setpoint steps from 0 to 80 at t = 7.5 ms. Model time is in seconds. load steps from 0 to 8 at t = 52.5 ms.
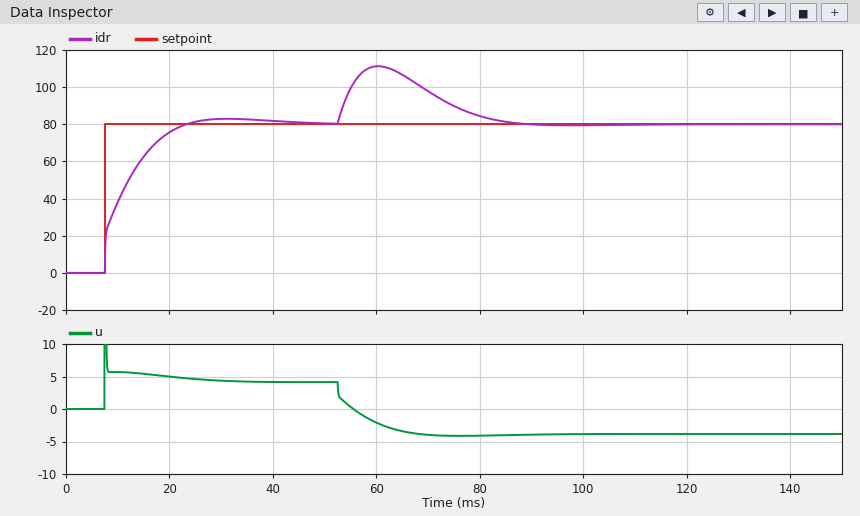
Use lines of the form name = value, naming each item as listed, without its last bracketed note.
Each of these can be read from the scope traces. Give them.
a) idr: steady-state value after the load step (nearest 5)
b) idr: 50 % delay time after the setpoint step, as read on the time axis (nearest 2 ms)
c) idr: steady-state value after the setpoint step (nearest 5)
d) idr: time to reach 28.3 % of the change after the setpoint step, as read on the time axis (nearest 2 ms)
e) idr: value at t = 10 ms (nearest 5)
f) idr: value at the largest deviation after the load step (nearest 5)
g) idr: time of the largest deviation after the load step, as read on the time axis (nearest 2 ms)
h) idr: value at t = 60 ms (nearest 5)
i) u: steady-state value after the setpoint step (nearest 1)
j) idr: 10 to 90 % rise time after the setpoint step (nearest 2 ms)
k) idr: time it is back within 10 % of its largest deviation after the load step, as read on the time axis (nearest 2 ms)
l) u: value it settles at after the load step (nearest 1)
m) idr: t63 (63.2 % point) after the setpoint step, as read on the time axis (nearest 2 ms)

idr: steady-state value after the load step = 80
idr: 50 % delay time after the setpoint step, as read on the time axis = 10 ms
idr: steady-state value after the setpoint step = 80
idr: time to reach 28.3 % of the change after the setpoint step, as read on the time axis = 8 ms
idr: value at t = 10 ms = 40
idr: value at the largest deviation after the load step = 110
idr: time of the largest deviation after the load step, as read on the time axis = 60 ms
idr: value at t = 60 ms = 110
u: steady-state value after the setpoint step = 4
idr: 10 to 90 % rise time after the setpoint step = 10 ms
idr: time it is back within 10 % of its largest deviation after the load step, as read on the time axis = 82 ms
u: value it settles at after the load step = -4
idr: t63 (63.2 % point) after the setpoint step, as read on the time axis = 12 ms
